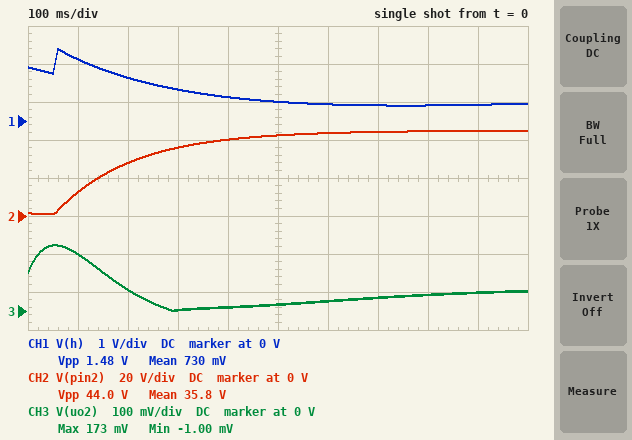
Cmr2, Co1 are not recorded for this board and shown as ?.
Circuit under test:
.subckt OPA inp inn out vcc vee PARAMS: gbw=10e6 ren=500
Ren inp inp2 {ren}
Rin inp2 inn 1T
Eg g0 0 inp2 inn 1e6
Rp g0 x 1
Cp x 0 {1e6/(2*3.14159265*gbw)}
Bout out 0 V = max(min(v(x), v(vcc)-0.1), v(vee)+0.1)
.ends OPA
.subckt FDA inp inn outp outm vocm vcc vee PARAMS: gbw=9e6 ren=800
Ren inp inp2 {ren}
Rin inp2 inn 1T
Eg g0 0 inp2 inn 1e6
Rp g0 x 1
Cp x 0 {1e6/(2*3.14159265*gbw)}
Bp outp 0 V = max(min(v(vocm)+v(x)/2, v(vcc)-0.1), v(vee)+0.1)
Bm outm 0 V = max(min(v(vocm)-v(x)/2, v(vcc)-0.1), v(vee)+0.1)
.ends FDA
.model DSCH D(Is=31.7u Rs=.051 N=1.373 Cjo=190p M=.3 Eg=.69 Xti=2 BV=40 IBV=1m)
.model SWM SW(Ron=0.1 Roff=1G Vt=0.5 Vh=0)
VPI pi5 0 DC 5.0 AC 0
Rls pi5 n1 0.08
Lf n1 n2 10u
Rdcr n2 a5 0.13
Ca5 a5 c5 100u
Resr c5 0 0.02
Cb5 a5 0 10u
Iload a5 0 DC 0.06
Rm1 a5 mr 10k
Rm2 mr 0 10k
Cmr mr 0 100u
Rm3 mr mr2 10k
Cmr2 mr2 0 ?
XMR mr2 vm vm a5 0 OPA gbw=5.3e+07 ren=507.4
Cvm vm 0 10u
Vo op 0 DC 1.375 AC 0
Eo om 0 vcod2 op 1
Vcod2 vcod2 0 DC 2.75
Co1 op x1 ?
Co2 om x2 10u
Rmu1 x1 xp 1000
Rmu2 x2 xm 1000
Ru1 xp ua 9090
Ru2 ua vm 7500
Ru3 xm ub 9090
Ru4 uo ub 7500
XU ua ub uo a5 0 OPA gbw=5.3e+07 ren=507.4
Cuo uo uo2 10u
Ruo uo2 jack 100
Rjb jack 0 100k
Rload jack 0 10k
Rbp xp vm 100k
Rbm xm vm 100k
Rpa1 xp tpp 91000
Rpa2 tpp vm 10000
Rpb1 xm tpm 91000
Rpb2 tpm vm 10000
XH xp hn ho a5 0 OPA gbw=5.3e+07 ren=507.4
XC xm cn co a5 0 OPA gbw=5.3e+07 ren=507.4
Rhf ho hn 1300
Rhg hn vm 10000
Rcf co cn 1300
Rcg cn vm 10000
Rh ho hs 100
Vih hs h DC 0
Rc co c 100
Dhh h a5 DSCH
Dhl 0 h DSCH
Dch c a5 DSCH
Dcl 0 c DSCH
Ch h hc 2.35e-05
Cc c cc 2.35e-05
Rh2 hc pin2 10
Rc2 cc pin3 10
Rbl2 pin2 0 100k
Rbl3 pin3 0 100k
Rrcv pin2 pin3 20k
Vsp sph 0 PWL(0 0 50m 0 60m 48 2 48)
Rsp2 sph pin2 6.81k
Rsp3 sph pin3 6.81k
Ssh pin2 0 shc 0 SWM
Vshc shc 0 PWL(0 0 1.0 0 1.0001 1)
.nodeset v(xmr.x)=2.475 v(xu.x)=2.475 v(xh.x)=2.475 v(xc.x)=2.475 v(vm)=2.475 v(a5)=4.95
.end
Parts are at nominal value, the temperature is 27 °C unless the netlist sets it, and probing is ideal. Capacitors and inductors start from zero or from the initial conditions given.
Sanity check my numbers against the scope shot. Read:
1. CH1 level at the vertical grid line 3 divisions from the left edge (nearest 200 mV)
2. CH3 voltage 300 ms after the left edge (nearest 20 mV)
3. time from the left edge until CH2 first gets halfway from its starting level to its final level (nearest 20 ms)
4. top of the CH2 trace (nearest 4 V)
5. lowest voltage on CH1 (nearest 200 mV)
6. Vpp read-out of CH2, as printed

800 mV
0 V
160 ms
44 V
400 mV
44.0 V
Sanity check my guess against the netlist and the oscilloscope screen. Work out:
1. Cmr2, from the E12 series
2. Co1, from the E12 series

150 µF
27 µF
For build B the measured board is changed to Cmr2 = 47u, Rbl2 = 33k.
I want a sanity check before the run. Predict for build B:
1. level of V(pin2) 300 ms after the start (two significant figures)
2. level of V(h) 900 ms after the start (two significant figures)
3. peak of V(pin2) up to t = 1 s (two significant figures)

34 V
830 mV
41 V
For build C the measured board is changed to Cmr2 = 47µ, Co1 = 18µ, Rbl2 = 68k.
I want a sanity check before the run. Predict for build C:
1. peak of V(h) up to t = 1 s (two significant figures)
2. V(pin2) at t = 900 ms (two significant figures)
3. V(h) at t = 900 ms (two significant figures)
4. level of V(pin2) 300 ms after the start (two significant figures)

1.8 V
44 V
890 mV
35 V
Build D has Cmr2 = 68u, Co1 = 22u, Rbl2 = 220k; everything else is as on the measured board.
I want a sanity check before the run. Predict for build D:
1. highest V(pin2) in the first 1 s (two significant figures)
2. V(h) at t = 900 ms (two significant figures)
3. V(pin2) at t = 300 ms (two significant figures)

46 V
690 mV
37 V
